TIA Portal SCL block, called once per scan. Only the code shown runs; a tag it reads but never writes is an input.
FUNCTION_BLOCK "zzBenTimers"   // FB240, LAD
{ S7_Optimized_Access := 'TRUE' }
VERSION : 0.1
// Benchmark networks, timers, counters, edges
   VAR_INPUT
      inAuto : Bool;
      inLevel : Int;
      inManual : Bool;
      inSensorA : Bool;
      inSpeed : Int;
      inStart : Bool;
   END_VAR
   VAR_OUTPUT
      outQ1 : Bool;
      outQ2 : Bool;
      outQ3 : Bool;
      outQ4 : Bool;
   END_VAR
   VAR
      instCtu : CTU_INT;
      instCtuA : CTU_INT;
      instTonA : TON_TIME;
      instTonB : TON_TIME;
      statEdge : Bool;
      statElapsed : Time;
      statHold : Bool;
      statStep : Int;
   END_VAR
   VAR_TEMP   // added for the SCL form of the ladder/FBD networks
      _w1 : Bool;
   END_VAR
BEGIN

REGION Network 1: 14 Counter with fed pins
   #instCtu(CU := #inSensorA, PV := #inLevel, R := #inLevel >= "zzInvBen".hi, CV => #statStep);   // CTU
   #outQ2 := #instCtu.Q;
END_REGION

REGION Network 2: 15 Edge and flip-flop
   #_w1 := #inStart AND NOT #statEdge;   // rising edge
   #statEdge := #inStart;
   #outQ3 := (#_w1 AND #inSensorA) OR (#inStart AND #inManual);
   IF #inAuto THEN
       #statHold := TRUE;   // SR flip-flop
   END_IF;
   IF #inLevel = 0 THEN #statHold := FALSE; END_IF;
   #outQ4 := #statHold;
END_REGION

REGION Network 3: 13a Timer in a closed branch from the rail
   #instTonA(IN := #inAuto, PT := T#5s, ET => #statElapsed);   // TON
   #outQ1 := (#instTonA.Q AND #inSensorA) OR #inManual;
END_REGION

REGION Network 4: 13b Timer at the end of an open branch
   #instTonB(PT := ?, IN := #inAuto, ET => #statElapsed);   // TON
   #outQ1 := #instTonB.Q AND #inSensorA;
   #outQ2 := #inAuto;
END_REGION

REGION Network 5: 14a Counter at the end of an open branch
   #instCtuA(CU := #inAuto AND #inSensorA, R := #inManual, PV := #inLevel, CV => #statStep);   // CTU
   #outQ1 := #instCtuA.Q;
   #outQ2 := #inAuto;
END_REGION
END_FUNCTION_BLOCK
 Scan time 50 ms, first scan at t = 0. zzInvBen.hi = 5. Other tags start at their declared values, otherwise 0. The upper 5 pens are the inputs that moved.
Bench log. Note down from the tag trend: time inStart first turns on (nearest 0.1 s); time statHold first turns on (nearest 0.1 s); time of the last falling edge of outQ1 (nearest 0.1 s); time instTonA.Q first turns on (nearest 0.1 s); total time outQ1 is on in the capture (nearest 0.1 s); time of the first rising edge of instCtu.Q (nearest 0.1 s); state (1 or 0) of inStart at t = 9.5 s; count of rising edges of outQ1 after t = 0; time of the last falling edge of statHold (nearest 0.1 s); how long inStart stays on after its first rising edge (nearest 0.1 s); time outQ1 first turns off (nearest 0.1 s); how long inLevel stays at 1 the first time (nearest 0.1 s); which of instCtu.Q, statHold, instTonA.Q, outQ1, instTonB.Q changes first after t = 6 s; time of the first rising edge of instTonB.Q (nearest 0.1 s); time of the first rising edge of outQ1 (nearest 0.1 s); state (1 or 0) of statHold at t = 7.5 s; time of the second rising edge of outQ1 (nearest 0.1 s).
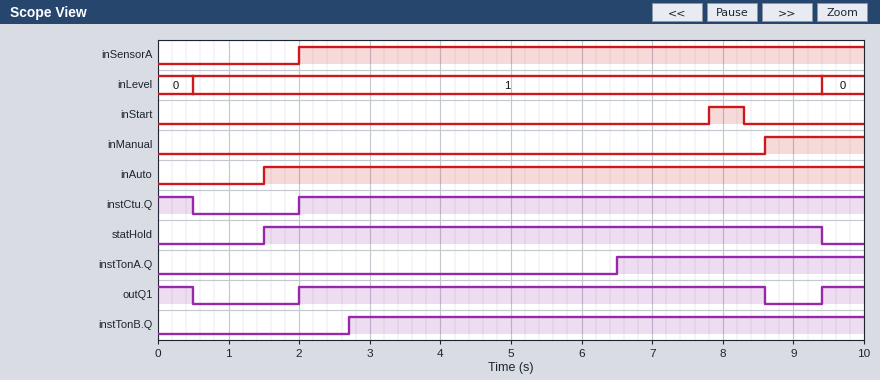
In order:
7.8 s
1.5 s
8.6 s
6.5 s
7.7 s
2.0 s
0
2
9.4 s
0.5 s
0.5 s
8.9 s
instTonA.Q
2.7 s
2.0 s
1
9.4 s
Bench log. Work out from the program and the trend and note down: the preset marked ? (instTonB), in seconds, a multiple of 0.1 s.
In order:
1.2 s
